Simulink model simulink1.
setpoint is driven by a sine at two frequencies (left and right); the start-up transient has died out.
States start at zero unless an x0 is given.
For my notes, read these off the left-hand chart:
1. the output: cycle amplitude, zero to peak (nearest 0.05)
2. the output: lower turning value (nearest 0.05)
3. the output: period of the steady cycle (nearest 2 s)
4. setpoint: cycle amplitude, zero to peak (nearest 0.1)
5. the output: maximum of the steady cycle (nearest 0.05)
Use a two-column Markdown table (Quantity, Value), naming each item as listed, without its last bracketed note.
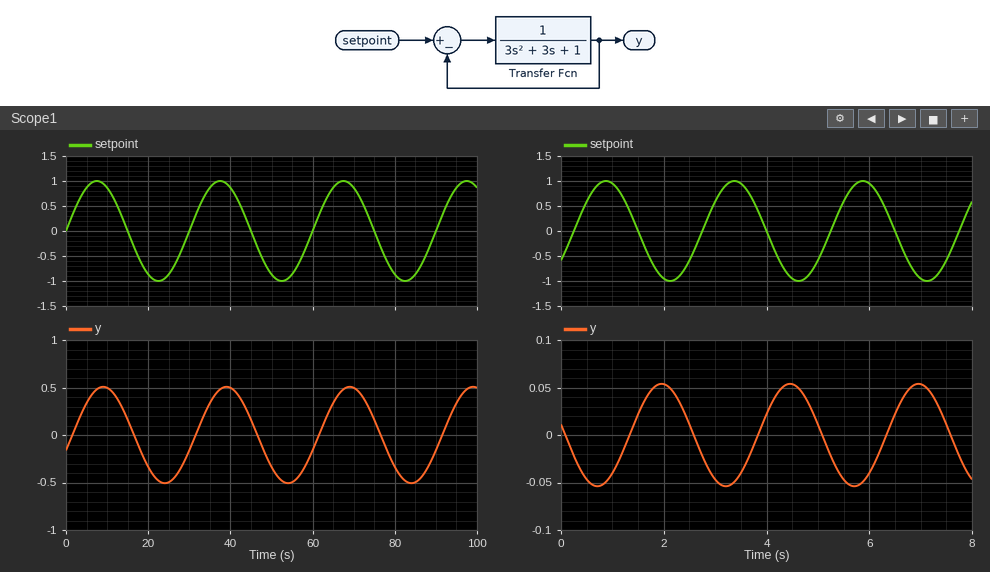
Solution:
| Quantity | Value |
|---|---|
| the output: cycle amplitude, zero to peak | 0.50 |
| the output: lower turning value | -0.50 |
| the output: period of the steady cycle | 30 s |
| setpoint: cycle amplitude, zero to peak | 1.0 |
| the output: maximum of the steady cycle | 0.50 |
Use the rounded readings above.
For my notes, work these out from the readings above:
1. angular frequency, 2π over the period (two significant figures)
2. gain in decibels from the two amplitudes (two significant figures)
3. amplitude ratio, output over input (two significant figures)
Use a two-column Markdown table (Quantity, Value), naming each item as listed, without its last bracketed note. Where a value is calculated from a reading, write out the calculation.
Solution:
| Quantity | Value |
|---|---|
| angular frequency, 2π over the period | 2π / 30 = 0.21 rad/s |
| gain in decibels from the two amplitudes | 20 log10(0.5 / 1) = -6.0 dB |
| amplitude ratio, output over input | 0.5 / 1 = 0.50 |
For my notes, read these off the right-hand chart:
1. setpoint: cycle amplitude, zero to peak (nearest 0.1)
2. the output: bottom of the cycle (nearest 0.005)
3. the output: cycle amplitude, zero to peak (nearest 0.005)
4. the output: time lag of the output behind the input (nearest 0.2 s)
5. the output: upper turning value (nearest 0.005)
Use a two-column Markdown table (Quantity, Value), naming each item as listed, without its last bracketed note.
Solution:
| Quantity | Value |
|---|---|
| setpoint: cycle amplitude, zero to peak | 1.0 |
| the output: bottom of the cycle | -0.055 |
| the output: cycle amplitude, zero to peak | 0.055 |
| the output: time lag of the output behind the input | 1.0 s |
| the output: upper turning value | 0.055 |
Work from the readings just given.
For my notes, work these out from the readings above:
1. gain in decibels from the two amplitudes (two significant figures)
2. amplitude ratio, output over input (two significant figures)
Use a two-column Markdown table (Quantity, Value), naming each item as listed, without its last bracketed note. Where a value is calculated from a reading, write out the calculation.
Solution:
| Quantity | Value |
|---|---|
| gain in decibels from the two amplitudes | 20 log10(0.055 / 1) = -25 dB |
| amplitude ratio, output over input | 0.055 / 1 = 0.055 |
